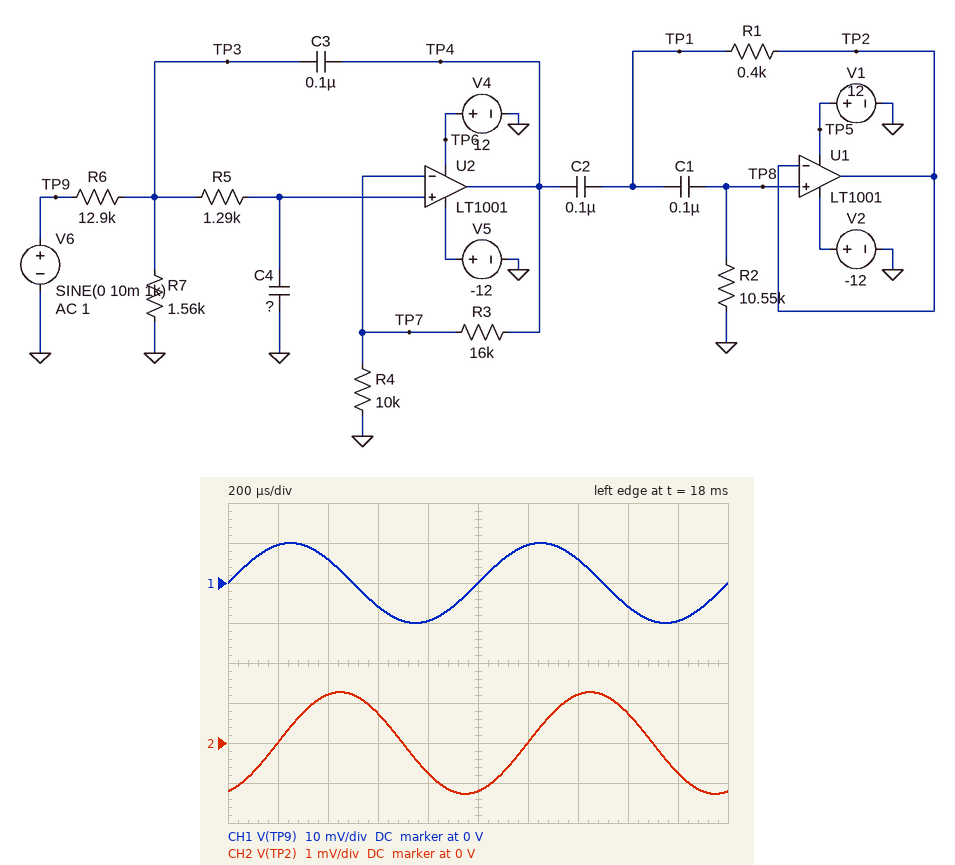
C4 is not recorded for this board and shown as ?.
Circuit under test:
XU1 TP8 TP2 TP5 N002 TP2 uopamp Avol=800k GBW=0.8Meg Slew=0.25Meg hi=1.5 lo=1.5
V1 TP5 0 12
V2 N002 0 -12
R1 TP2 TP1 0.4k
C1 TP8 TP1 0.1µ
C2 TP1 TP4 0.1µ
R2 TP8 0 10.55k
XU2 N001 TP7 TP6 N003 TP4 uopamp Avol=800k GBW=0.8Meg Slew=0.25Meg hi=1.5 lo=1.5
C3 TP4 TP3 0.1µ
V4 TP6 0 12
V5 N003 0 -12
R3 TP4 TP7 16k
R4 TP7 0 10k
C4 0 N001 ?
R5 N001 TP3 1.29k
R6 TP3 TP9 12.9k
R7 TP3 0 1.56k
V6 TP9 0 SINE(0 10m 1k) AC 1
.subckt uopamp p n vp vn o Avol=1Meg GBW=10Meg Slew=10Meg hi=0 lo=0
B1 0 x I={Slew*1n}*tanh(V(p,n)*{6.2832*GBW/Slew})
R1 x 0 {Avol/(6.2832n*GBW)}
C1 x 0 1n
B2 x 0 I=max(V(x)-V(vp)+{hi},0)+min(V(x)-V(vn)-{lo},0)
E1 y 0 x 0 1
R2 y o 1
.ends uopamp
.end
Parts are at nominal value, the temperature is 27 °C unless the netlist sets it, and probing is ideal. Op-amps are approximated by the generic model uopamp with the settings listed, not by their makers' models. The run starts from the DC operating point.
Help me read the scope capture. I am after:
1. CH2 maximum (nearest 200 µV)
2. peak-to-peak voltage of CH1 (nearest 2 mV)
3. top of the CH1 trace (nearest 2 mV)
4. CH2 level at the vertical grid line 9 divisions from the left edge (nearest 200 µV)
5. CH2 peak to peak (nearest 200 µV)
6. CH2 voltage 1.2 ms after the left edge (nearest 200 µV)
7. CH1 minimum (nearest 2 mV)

1.2 mV
20 mV
10 mV
-800 µV
2.6 mV
0 V
-10 mV
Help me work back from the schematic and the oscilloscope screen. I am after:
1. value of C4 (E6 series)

330 nF
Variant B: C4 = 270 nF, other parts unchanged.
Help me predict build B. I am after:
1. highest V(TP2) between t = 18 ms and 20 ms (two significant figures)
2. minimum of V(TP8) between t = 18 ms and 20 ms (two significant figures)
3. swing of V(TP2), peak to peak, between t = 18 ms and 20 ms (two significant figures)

1.7 mV
-1.7 mV
3.4 mV
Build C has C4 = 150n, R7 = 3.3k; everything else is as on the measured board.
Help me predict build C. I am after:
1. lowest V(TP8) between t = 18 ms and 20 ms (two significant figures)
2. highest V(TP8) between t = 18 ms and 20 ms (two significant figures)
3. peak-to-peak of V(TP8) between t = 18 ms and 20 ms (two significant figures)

-7.2 mV
7.2 mV
14 mV
